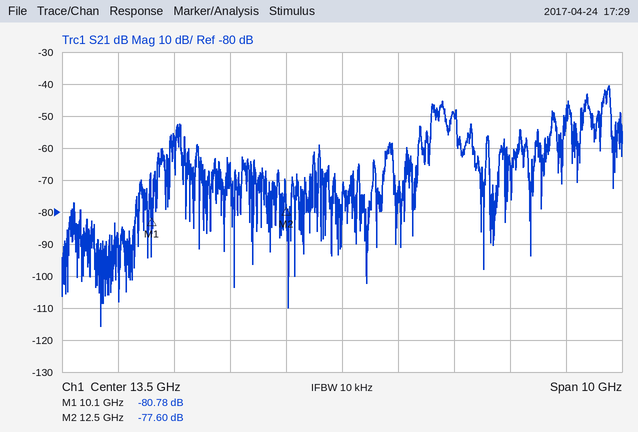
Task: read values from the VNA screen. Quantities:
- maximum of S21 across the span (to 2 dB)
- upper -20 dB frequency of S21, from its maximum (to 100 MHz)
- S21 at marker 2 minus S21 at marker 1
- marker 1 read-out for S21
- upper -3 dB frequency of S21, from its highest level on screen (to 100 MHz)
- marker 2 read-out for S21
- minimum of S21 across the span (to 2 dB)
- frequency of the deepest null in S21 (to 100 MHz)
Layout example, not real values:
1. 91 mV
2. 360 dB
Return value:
1. -40 dB
2. 18.3 GHz
3. 3.18 dB
4. -80.78 dB
5. 18.3 GHz
6. -77.60 dB
7. -116 dB
8. 9.2 GHz
